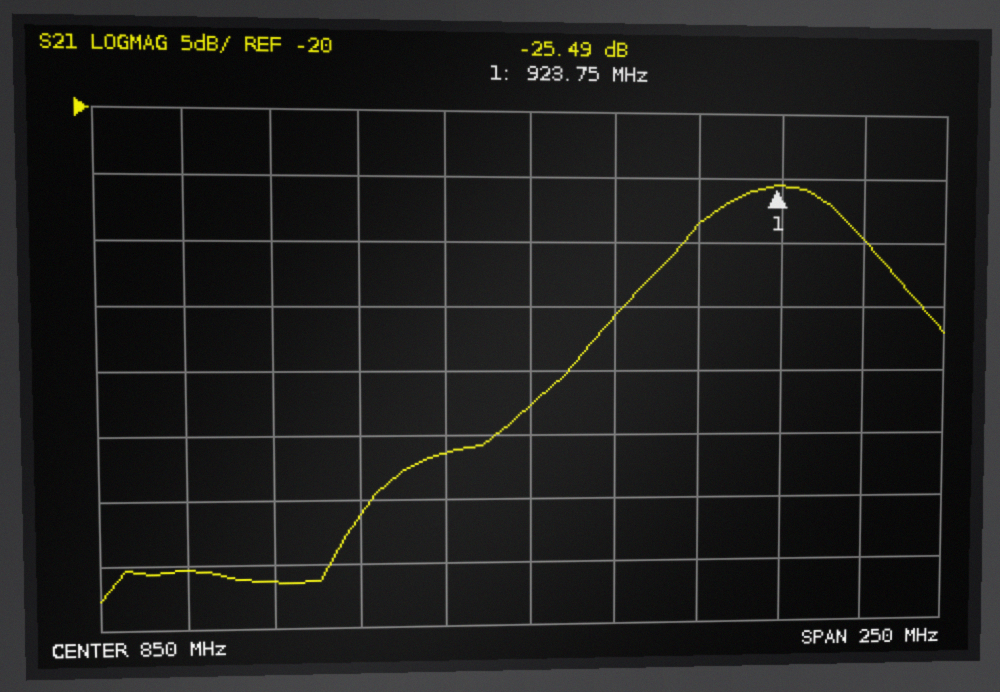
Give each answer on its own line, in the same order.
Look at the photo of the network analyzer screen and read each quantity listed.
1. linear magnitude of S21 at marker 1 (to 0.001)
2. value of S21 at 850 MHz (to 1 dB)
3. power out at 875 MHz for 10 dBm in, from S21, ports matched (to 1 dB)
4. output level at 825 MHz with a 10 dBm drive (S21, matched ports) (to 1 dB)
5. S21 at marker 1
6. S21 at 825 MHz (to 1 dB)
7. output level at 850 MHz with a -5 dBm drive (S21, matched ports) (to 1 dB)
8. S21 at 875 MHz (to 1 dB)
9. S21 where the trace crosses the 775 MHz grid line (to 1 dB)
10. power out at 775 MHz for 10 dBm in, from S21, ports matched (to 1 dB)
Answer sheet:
0.053
-43 dB
-26 dBm
-36 dBm
-25.49 dB
-46 dB
-48 dBm
-36 dB
-56 dB
-46 dBm
